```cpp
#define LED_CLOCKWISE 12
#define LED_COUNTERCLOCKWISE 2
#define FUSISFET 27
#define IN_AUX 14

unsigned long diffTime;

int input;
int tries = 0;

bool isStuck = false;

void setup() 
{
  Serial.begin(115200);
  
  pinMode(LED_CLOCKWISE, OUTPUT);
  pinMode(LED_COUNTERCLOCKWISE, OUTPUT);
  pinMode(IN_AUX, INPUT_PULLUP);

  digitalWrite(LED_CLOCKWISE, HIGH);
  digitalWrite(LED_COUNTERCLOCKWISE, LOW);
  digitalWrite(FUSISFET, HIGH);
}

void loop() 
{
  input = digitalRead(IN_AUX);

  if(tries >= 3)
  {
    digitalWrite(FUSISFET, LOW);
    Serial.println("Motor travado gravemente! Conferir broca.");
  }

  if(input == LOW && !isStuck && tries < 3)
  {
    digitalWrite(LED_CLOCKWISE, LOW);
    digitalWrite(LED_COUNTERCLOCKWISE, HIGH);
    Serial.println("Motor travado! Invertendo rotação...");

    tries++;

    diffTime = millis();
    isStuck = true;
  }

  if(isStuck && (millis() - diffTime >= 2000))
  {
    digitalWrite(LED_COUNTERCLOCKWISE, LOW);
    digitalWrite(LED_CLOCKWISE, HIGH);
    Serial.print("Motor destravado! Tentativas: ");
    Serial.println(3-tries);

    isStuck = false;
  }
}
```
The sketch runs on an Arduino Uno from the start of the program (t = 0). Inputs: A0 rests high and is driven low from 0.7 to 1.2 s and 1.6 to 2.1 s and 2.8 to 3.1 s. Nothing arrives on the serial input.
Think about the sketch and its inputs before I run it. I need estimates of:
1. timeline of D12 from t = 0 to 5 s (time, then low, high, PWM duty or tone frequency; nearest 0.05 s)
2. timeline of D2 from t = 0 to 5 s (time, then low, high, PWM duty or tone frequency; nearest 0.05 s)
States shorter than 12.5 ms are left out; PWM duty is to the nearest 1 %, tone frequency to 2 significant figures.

0 s high; 0.7 s low; 2.7 s high; 2.8 s low; 4.8 s high
0 s low; 0.7 s high; 2.7 s low; 2.8 s high; 4.8 s low
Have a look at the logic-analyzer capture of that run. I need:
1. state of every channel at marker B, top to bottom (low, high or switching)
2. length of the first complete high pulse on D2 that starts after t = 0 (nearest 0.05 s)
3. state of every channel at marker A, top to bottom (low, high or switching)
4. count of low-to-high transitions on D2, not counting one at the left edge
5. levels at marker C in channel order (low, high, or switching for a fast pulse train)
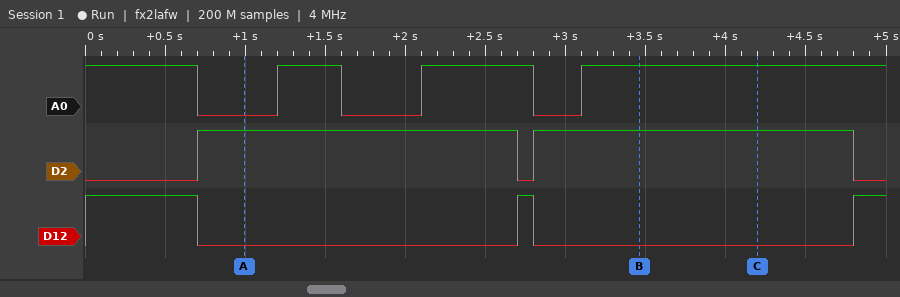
A0 high, D2 high, D12 low
2.00 s
A0 low, D2 high, D12 low
2
A0 high, D2 high, D12 low
